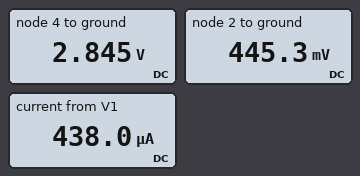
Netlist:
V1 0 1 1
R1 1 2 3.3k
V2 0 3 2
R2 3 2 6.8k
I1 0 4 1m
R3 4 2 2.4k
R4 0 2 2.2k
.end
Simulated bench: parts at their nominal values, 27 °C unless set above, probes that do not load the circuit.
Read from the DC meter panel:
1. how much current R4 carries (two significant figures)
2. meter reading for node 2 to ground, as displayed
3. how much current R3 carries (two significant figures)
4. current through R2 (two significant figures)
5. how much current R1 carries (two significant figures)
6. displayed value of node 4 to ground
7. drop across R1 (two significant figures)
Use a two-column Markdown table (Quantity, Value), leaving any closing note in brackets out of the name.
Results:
| Quantity | Value |
|---|---|
| how much current R4 carries | 200 µA |
| meter reading for node 2 to ground, as displayed | 445.3 mV |
| how much current R3 carries | 1.0 mA |
| current through R2 | 360 µA |
| how much current R1 carries | 440 µA |
| displayed value of node 4 to ground | 2.845 V |
| drop across R1 | 1.4 V |
